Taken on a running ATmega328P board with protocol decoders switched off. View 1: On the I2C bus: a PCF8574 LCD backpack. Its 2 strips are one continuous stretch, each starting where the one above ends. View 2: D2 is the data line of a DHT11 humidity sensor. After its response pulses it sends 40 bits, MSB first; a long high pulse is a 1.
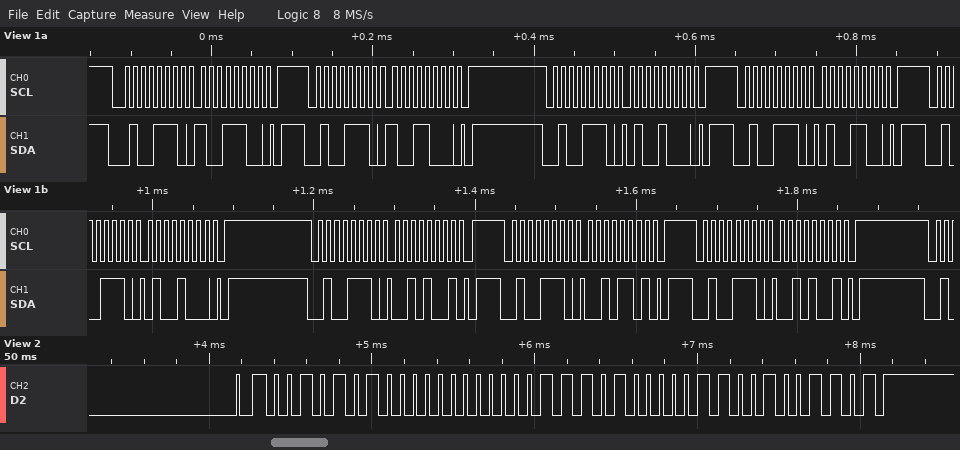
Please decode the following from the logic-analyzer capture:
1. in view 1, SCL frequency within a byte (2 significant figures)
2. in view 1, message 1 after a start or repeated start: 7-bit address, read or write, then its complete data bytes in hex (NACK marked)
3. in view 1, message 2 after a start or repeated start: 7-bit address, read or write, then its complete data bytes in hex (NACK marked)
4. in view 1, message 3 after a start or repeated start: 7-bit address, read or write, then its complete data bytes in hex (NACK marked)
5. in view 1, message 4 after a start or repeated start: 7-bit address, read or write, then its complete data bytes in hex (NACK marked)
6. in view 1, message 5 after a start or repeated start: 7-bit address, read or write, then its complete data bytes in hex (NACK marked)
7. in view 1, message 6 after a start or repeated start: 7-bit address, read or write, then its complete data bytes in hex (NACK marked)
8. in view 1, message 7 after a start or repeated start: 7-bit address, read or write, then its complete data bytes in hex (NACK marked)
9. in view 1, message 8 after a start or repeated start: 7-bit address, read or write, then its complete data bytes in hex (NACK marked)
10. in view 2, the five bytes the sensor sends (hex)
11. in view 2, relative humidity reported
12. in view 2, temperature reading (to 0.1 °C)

100 kHz
0x27 write: 9C
0x27 write: 98
0x27 write: 48
0x27 write: 4C
0x27 write: 48
0x27 write: 29
0x27 write: 2D
0x27 write: 29
2A 00 1D 06 4D
42 %
29.6 °C
